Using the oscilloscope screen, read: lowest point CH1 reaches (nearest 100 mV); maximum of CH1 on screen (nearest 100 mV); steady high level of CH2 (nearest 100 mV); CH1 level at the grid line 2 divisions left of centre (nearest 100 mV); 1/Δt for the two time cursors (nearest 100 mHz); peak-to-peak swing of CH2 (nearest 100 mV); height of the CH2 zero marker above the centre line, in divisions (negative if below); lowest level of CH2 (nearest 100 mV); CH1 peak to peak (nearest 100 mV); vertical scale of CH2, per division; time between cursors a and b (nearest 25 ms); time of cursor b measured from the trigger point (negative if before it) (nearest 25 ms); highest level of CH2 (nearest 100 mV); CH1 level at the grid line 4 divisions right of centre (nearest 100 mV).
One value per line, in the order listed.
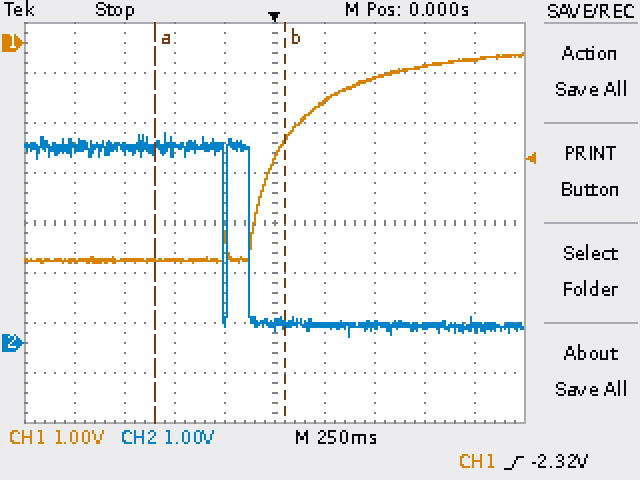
-4.4 V
-200 mV
3.9 V
-4.3 V
1.5 Hz
4.1 V
-2.4 div
100 mV
4.2 V
1 V
650 ms
+50 ms
4.2 V
-300 mV
